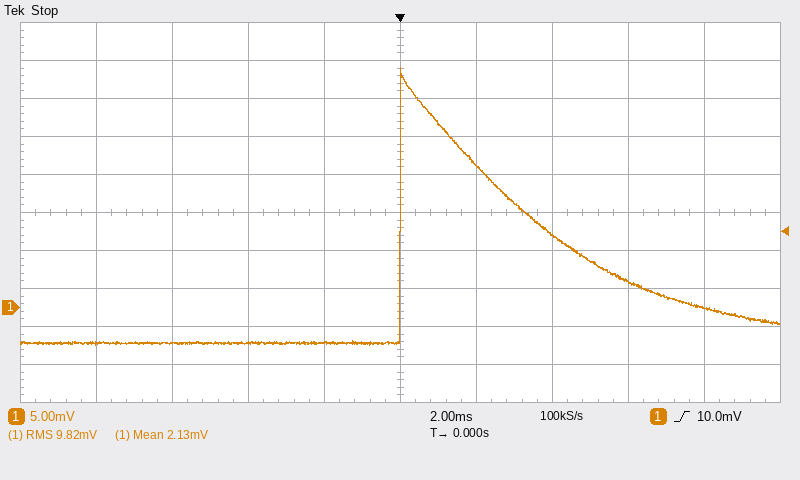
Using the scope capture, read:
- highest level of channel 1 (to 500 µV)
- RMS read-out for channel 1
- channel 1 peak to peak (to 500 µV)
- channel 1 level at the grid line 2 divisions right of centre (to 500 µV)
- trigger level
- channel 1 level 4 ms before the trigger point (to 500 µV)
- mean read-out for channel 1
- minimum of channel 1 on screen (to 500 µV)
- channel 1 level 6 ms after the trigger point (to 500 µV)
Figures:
31.5 mV
9.82 mV
36.5 mV
9.5 mV
10.0 mV
-4.5 mV
2.13 mV
-5.0 mV
3.5 mV
